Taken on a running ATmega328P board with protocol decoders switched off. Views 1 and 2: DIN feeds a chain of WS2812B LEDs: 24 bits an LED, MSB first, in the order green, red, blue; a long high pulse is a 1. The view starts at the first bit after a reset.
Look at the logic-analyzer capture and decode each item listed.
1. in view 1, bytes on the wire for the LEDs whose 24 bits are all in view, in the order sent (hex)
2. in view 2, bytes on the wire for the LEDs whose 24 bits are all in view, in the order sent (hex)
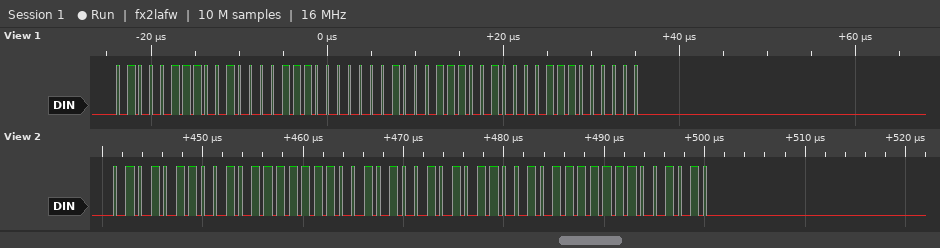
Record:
47 21 C0 47 21 C0
56 5F CA 56 5F CA
